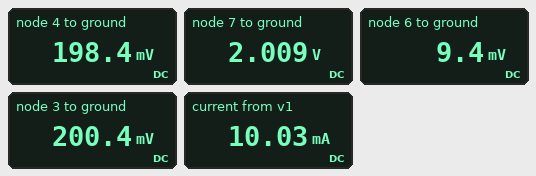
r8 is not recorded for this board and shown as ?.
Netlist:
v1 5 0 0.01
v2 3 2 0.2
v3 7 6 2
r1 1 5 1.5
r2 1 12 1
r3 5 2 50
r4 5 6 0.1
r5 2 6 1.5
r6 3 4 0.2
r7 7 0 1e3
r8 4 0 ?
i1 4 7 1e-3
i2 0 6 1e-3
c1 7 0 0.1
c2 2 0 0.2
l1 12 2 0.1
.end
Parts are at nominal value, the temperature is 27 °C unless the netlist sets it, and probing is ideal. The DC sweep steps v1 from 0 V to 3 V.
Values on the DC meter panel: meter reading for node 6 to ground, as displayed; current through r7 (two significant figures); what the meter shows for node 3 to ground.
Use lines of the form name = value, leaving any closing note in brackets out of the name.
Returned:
meter reading for node 6 to ground, as displayed = 9.4 mV
current through r7 = 2.0 mA
what the meter shows for node 3 to ground = 200.4 mV
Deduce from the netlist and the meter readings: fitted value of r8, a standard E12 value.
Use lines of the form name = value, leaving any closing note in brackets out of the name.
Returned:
fitted value of r8, a standard E12 value = 22 Ω
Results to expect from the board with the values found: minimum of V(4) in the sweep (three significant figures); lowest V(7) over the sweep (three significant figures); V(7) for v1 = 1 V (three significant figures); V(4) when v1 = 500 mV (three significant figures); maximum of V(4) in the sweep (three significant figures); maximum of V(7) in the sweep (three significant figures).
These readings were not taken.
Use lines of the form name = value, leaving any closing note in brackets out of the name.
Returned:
minimum of V(4) in the sweep = 189 mV
lowest V(7) over the sweep = 2.00 V
V(7) for v1 = 1 V = 3.00 V
V(4) when v1 = 500 mV = 664 mV
maximum of V(4) in the sweep = 3.04 V
maximum of V(7) in the sweep = 4.99 V
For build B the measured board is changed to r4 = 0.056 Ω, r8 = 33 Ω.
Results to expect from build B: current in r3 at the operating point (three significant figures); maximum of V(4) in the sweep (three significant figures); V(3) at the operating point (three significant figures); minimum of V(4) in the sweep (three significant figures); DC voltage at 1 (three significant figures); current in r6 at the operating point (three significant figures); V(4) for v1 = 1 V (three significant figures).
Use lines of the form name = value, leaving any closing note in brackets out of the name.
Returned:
current in r3 at the operating point = 134 µA
maximum of V(4) in the sweep = 3.09 V
V(3) at the operating point = 203 mV
minimum of V(4) in the sweep = 192 mV
DC voltage at 1 = 5.98 mV
current in r6 at the operating point = 7.12 mA
V(4) for v1 = 1 V = 1.16 V
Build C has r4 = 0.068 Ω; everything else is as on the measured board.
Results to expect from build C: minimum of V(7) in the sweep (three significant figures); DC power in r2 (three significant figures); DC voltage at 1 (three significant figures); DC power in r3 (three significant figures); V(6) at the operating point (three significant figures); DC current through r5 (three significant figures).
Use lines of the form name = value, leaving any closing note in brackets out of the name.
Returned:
minimum of V(7) in the sweep = 2.00 V
DC power in r2 = 14.4 µW
DC voltage at 1 = 4.31 mV
DC power in r3 = 1.80 µW
V(6) at the operating point = 9.59 mV
DC current through r5 = 6.04 mA
